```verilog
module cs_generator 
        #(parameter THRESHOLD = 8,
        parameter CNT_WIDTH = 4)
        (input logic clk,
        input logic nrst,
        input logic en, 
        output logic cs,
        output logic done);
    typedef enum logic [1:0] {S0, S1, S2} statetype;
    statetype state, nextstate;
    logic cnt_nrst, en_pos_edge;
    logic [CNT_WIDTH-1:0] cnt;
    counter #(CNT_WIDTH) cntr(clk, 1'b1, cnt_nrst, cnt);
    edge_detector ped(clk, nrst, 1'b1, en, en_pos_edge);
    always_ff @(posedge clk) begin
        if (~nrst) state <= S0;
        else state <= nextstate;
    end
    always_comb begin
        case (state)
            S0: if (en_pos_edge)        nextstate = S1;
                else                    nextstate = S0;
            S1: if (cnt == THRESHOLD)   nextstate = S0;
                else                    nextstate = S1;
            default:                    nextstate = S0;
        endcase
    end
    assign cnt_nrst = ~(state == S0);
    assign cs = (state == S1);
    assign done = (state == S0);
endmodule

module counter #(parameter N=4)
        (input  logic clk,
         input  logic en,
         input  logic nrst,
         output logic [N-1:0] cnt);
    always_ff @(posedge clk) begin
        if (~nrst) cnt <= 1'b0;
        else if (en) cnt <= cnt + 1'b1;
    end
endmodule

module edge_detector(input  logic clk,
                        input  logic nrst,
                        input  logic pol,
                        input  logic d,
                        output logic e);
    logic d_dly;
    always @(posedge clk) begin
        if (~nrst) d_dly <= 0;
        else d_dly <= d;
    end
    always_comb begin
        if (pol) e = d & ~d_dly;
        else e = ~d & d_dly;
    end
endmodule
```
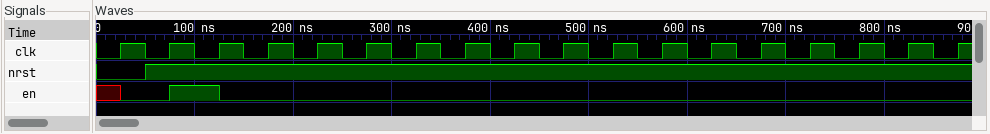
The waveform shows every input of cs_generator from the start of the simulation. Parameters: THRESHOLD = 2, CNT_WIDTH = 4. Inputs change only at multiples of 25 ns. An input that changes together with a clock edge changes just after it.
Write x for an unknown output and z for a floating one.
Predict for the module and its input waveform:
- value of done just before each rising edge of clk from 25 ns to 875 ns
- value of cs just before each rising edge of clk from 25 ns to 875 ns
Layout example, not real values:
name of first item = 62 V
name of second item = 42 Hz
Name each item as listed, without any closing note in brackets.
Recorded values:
value of done just before each rising edge of clk from 25 ns to 875 ns = x 1 1 0 0 0 1 1 1 1 1 1 1 1 1 1 1 1
value of cs just before each rising edge of clk from 25 ns to 875 ns = x 0 0 1 1 1 0 0 0 0 0 0 0 0 0 0 0 0
